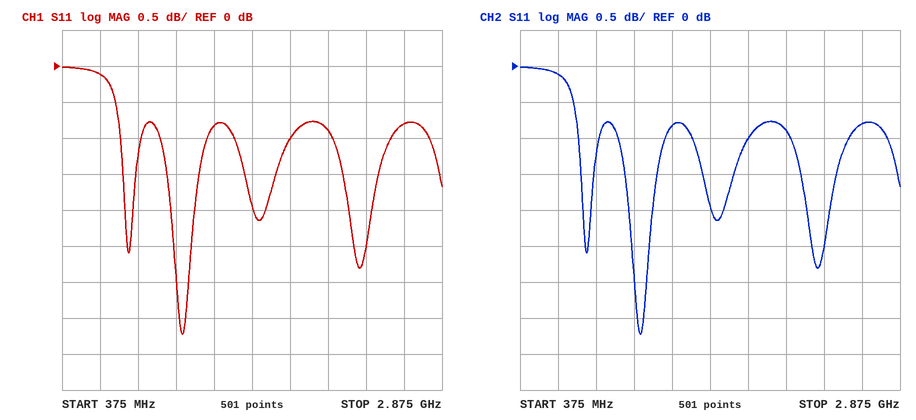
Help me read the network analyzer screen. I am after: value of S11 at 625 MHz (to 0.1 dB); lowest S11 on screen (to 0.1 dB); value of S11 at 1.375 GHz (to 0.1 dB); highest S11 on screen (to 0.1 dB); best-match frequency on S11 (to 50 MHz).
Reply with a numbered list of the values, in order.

1. -0.1 dB
2. -3.7 dB
3. -0.8 dB
4. 0.0 dB
5. 1.15 GHz
